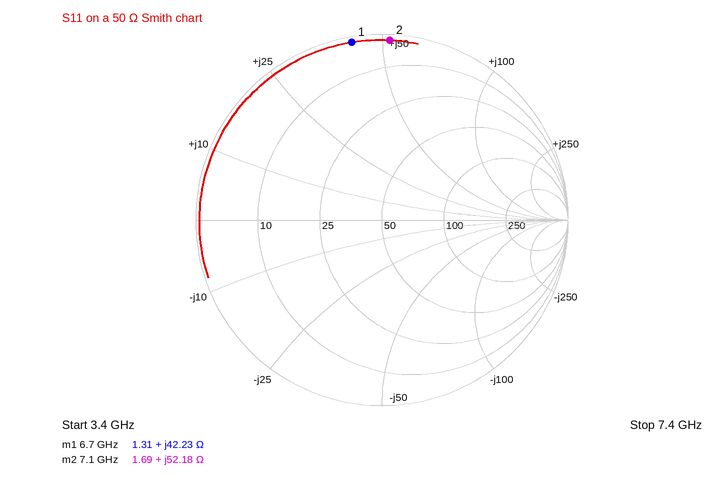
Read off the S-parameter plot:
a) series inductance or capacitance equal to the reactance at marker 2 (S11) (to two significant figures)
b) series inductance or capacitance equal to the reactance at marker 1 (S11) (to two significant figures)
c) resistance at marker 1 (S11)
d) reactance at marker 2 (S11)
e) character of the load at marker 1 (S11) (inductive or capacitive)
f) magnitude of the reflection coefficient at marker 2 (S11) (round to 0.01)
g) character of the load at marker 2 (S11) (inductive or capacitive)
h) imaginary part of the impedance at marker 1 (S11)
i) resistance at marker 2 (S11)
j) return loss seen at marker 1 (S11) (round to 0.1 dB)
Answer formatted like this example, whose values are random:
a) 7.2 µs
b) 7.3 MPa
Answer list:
a) 1.2 nH
b) 1.0 nH
c) 1.31 Ω
d) +52.18 Ω
e) inductive
f) 0.97
g) inductive
h) +42.23 Ω
i) 1.69 Ω
j) 0.3 dB
